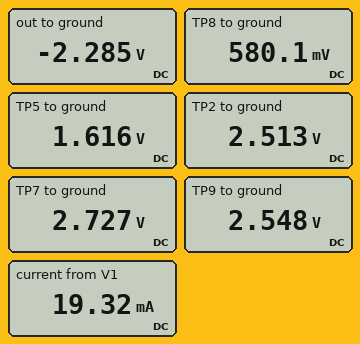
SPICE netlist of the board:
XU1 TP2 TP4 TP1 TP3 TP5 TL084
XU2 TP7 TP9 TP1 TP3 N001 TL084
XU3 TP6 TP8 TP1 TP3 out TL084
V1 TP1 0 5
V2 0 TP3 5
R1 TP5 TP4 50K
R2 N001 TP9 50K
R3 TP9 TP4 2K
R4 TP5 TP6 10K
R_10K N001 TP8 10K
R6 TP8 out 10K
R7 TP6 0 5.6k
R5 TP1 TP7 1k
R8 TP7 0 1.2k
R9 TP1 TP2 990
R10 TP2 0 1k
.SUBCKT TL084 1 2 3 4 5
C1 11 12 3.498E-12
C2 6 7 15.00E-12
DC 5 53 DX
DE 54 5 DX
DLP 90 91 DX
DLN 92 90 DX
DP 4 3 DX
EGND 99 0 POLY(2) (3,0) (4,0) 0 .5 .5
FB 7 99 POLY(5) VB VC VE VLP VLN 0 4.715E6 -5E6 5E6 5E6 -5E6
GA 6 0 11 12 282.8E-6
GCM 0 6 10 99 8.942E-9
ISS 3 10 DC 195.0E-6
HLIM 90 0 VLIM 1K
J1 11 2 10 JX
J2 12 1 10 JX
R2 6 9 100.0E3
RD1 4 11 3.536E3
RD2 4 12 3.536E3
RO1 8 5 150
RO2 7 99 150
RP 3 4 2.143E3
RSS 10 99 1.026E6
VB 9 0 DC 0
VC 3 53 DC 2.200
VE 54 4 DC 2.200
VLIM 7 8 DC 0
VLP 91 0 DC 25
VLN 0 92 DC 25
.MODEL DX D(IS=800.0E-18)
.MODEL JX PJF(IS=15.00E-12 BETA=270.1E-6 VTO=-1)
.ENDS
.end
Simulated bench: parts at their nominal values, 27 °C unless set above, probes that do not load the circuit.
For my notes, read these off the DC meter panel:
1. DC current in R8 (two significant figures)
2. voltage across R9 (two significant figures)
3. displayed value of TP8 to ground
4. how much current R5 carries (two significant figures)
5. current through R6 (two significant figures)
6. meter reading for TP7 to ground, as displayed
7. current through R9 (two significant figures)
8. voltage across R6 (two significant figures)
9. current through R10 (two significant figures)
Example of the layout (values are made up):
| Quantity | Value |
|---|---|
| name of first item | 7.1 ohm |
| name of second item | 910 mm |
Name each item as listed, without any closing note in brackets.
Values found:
| Quantity | Value |
|---|---|
| DC current in R8 | 2.3 mA |
| voltage across R9 | 2.5 V |
| displayed value of TP8 to ground | 580.1 mV |
| how much current R5 carries | 2.3 mA |
| current through R6 | 290 µA |
| meter reading for TP7 to ground, as displayed | 2.727 V |
| current through R9 | 2.5 mA |
| voltage across R6 | 2.9 V |
| current through R10 | 2.5 mA |
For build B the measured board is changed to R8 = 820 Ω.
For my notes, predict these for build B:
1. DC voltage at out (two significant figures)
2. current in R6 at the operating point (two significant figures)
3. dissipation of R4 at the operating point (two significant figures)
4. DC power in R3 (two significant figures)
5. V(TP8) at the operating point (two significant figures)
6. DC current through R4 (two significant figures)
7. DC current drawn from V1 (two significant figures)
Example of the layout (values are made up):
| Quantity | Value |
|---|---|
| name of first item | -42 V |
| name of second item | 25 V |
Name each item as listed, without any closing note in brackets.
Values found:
| Quantity | Value |
|---|---|
| DC voltage at out | 1.4 V |
| current in R6 at the operating point | 14 µA |
| dissipation of R4 at the operating point | 490 µW |
| DC power in R3 | 1.1 µW |
| V(TP8) at the operating point | 1.2 V |
| DC current through R4 | 220 µA |
| DC current drawn from V1 | 20 mA |
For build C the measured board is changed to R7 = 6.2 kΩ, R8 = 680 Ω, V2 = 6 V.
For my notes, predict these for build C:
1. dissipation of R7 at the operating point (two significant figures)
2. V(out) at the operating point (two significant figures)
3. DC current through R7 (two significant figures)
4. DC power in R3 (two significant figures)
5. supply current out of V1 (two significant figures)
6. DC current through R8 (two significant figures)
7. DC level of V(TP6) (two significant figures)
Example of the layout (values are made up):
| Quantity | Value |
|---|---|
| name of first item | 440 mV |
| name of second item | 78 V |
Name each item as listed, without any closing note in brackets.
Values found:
| Quantity | Value |
|---|---|
| dissipation of R7 at the operating point | 280 µW |
| V(out) at the operating point | 2.0 V |
| DC current through R7 | 210 µA |
| DC power in R3 | 1.5 µW |
| supply current out of V1 | 21 mA |
| DC current through R8 | 3.0 mA |
| DC level of V(TP6) | 1.3 V |
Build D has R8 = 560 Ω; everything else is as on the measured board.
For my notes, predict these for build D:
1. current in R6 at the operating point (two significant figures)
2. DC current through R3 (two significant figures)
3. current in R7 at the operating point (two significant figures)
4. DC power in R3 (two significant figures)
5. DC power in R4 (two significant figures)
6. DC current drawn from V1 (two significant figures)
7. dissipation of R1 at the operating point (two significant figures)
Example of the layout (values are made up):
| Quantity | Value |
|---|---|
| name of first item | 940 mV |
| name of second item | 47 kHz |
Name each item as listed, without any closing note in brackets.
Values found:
| Quantity | Value |
|---|---|
| current in R6 at the operating point | 110 µA |
| DC current through R3 | 32 µA |
| current in R7 at the operating point | 220 µA |
| DC power in R3 | 2.1 µW |
| DC power in R4 | 500 µW |
| DC current drawn from V1 | 20 mA |
| dissipation of R1 at the operating point | 52 µW |
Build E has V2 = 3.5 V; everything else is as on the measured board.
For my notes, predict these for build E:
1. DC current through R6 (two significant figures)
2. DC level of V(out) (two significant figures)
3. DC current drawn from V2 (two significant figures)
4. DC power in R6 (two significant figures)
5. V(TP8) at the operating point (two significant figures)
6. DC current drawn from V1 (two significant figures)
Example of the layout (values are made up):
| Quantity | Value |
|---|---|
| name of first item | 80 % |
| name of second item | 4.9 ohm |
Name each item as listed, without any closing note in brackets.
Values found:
| Quantity | Value |
|---|---|
| DC current through R6 | 270 µA |
| DC level of V(out) | -1.9 V |
| DC current drawn from V2 | 12 mA |
| DC power in R6 | 730 µW |
| V(TP8) at the operating point | 750 mV |
| DC current drawn from V1 | 17 mA |
